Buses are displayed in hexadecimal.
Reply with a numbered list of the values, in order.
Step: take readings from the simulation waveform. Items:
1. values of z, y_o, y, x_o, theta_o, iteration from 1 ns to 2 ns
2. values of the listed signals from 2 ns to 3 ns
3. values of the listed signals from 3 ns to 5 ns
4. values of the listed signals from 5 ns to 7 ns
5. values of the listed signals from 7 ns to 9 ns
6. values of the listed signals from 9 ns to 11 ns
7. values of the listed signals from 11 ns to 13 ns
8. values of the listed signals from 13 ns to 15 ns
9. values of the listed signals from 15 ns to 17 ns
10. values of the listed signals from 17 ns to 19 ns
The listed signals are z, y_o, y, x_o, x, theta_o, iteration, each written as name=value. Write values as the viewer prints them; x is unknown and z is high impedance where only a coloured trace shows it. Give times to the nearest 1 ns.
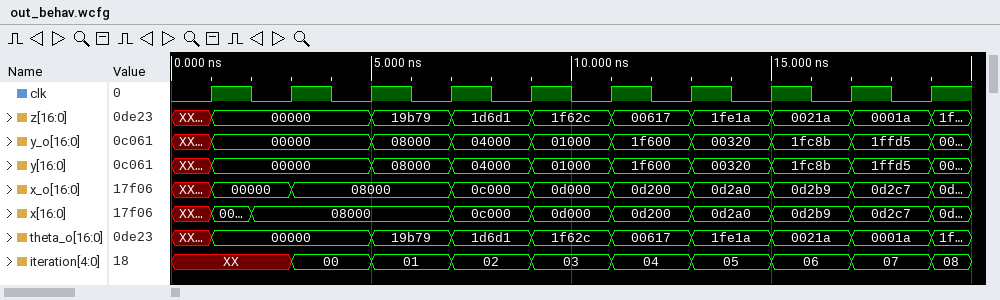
1. z=00000, y_o=00000, y=00000, x_o=00000, theta_o=00000, iteration=XX
2. z=00000, y_o=00000, y=00000, x_o=00000, x=08000, theta_o=00000, iteration=XX
3. z=00000, y_o=00000, y=00000, x_o=08000, x=08000, theta_o=00000, iteration=00
4. z=19b79, y_o=08000, y=08000, x_o=08000, x=08000, theta_o=19b79, iteration=01
5. z=1d6d1, y_o=04000, y=04000, x_o=0c000, x=0c000, theta_o=1d6d1, iteration=02
6. z=1f62c, y_o=01000, y=01000, x_o=0d000, x=0d000, theta_o=1f62c, iteration=03
7. z=00617, y_o=1f600, y=1f600, x_o=0d200, x=0d200, theta_o=00617, iteration=04
8. z=1fe1a, y_o=00320, y=00320, x_o=0d2a0, x=0d2a0, theta_o=1fe1a, iteration=05
9. z=0021a, y_o=1fc8b, y=1fc8b, x_o=0d2b9, x=0d2b9, theta_o=0021a, iteration=06
10. z=0001a, y_o=1ffd5, y=1ffd5, x_o=0d2c7, x=0d2c7, theta_o=0001a, iteration=07
